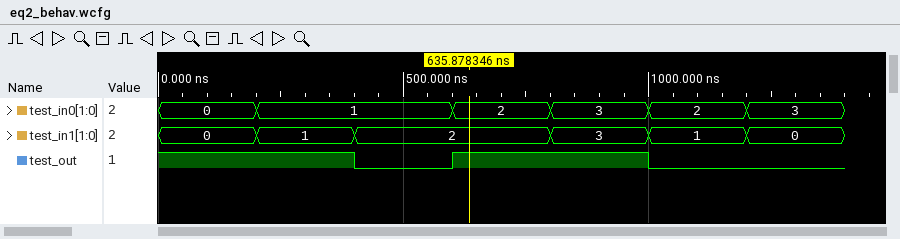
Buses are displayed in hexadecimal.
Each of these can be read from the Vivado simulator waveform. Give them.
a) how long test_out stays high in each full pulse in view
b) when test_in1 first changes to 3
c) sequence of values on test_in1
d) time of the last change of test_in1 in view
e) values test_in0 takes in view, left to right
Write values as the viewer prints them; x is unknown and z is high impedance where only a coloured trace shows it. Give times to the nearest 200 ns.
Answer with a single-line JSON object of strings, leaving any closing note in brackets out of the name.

{"how long test_out stays high in each full pulse in view": "400 ns", "when test_in1 first changes to 3": "800 ns", "sequence of values on test_in1": "0, 1, 2, 3, 1, 0", "time of the last change of test_in1 in view": "1200 ns", "values test_in0 takes in view, left to right": "0, 1, 2, 3, 2, 3"}
